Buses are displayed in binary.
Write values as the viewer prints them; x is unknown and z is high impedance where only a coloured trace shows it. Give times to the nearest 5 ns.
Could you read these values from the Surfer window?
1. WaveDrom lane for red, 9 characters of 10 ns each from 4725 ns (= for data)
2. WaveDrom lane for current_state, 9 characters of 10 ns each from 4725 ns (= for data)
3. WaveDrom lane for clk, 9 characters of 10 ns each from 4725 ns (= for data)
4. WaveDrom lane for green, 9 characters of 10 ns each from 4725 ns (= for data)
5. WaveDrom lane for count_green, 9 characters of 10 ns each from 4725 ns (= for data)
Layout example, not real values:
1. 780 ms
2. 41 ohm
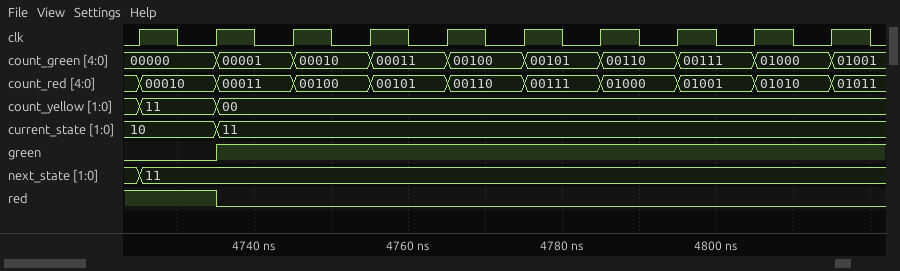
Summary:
1. {name: 'red', wave: '10.......'}
2. {name: 'current_state', wave: '==.......', data: '10 11'}
3. {name: 'clk', wave: 'p........'}
4. {name: 'green', wave: '01.......'}
5. {name: 'count_green', wave: '=========', data: '00000 00001 00010 00011 00100 00101 00110 00111 01000'}
